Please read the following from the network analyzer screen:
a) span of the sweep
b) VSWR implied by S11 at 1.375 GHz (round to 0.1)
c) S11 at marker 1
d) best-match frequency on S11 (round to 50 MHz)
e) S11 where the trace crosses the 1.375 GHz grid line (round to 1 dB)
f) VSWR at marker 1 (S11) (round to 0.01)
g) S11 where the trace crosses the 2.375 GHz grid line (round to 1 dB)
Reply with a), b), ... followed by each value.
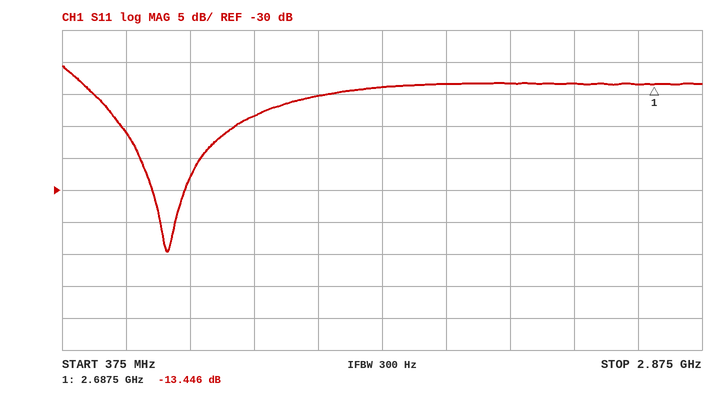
a) 2.5 GHz
b) 1.4
c) -13.446 dB
d) 800 MHz
e) -15 dB
f) 1.54
g) -13 dB
